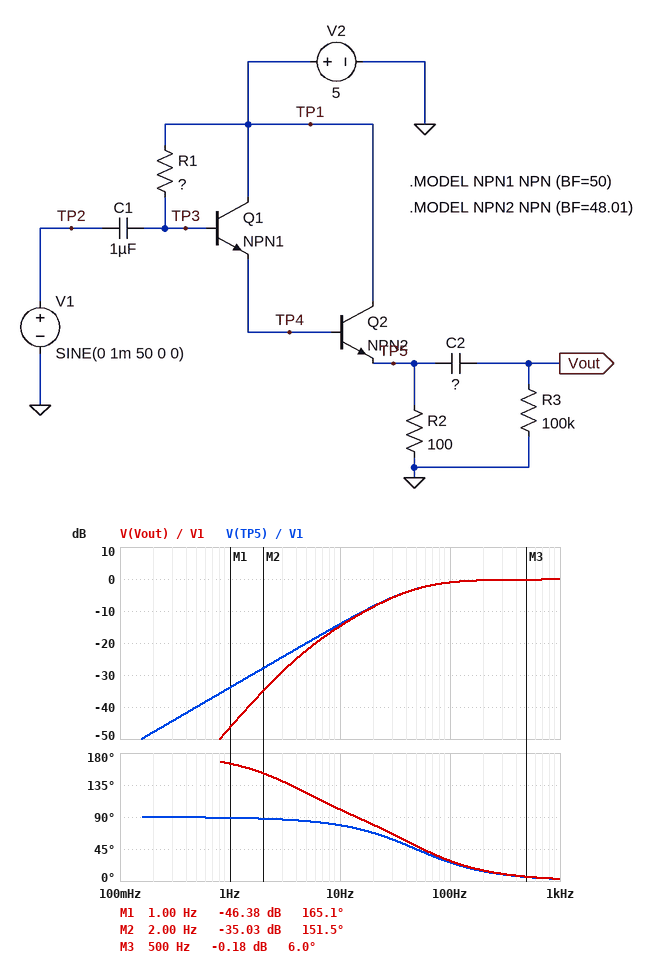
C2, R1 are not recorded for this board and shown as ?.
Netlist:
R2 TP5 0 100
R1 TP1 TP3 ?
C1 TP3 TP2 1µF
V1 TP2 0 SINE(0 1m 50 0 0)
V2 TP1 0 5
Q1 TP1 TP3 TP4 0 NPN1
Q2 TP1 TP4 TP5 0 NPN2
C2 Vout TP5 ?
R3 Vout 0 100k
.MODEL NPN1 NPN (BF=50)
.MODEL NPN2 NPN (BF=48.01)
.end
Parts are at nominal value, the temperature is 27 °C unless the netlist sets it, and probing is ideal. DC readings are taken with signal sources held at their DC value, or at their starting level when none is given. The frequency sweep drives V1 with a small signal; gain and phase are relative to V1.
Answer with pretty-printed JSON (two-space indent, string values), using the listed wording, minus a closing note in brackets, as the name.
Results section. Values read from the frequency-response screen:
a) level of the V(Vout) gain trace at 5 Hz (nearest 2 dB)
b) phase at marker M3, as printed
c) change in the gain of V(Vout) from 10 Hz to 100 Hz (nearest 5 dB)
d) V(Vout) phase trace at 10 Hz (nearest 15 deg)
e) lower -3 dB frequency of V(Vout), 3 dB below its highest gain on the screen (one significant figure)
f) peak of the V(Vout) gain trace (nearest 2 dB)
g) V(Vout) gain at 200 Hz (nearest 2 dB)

{
  "level of the V(Vout) gain trace at 5 Hz": "-22 dB",
  "phase at marker M3, as printed": "6.0 deg",
  "change in the gain of V(Vout) from 10 Hz to 100 Hz": "15 dB",
  "V(Vout) phase trace at 10 Hz": "105 deg",
  "lower -3 dB frequency of V(Vout), 3 dB below its highest gain on the screen": "50 Hz",
  "peak of the V(Vout) gain trace": "0 dB",
  "V(Vout) gain at 200 Hz": "0 dB"
}
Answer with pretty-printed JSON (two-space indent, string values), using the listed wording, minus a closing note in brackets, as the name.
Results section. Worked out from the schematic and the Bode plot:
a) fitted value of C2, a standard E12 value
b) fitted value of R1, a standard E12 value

{
  "fitted value of C2, a standard E12 value": "390 nF",
  "fitted value of R1, a standard E12 value": "3.3 kΩ"
}
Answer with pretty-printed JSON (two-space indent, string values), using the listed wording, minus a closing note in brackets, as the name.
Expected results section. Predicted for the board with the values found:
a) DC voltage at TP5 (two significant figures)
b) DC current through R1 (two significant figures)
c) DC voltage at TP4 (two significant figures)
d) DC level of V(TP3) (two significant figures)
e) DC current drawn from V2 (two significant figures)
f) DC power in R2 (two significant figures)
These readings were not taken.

{
  "DC voltage at TP5": "3.3 V",
  "DC current through R1": "13 µA",
  "DC voltage at TP4": "4.2 V",
  "DC level of V(TP3)": "5.0 V",
  "DC current drawn from V2": "33 mA",
  "DC power in R2": "110 mW"
}
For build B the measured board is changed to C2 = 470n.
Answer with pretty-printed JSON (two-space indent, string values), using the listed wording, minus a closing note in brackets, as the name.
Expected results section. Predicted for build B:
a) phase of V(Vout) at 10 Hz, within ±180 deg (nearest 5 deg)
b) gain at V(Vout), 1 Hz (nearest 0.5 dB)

{
  "phase of V(Vout) at 10 Hz, within ±180 deg": "95 deg",
  "gain at V(Vout), 1 Hz": "-45.0 dB"
}
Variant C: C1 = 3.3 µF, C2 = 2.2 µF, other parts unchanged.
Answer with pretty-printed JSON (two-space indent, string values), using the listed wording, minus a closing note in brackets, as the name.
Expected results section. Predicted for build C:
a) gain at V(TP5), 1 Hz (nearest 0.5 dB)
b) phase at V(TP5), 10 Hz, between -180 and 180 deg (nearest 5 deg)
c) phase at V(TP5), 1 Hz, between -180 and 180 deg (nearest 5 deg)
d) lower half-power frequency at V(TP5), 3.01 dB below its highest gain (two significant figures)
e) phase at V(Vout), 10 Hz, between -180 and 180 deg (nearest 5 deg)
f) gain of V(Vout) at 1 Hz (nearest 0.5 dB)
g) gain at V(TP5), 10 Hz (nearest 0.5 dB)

{
  "gain at V(TP5), 1 Hz": "-23.5 dB",
  "phase at V(TP5), 10 Hz, between -180 and 180 deg": "55 deg",
  "phase at V(TP5), 1 Hz, between -180 and 180 deg": "85 deg",
  "lower half-power frequency at V(TP5), 3.01 dB below its highest gain": "15 Hz",
  "phase at V(Vout), 10 Hz, between -180 and 180 deg": "60 deg",
  "gain of V(Vout) at 1 Hz": "-25.5 dB",
  "gain at V(TP5), 10 Hz": "-5.0 dB"
}
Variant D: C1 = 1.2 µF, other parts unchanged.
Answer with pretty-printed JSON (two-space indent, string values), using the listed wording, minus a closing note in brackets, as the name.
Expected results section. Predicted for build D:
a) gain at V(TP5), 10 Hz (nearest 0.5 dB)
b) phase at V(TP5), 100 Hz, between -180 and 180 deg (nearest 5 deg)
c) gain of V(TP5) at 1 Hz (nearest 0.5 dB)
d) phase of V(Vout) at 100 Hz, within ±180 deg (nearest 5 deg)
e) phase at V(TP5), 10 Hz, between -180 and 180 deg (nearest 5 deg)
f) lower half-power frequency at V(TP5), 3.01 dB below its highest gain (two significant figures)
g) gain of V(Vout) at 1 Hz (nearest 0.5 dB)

{
  "gain at V(TP5), 10 Hz": "-12.5 dB",
  "phase at V(TP5), 100 Hz, between -180 and 180 deg": "20 deg",
  "gain of V(TP5) at 1 Hz": "-32.5 dB",
  "phase of V(Vout) at 100 Hz, within ±180 deg": "25 deg",
  "phase at V(TP5), 10 Hz, between -180 and 180 deg": "75 deg",
  "lower half-power frequency at V(TP5), 3.01 dB below its highest gain": "41 Hz",
  "gain of V(Vout) at 1 Hz": "-45.0 dB"
}
